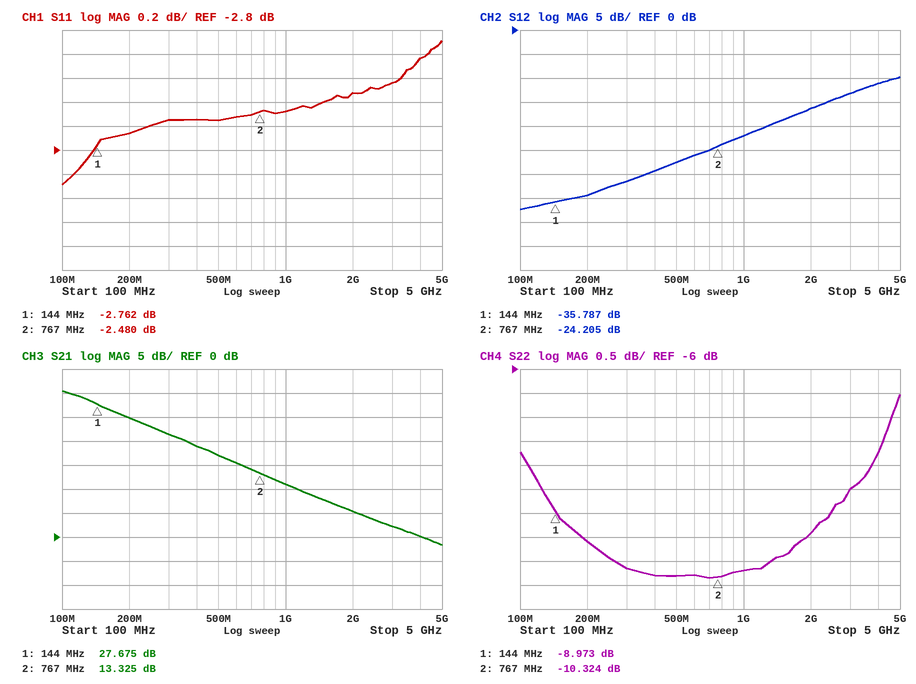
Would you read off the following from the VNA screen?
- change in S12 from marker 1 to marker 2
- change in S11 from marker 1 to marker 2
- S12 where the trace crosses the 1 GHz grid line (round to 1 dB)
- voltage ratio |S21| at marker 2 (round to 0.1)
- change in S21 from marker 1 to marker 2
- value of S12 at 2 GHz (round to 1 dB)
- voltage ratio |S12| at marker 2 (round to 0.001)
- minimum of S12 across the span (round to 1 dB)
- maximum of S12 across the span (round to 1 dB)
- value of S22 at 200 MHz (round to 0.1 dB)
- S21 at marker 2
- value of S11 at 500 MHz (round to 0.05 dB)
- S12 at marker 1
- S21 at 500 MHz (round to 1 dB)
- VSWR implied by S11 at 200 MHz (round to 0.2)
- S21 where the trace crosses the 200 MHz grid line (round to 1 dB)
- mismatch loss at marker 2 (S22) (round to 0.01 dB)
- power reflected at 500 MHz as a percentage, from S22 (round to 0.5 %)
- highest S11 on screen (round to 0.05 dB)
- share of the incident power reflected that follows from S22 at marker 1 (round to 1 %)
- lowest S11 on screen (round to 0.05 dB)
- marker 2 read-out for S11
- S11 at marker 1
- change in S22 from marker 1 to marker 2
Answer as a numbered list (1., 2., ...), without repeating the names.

1. 11.582 dB
2. 0.282 dB
3. -22 dB
4. 4.6
5. -14.350 dB
6. -16 dB
7. 0.062
8. -37 dB
9. -10 dB
10. -9.6 dB
11. 13.325 dB
12. -2.55 dB
13. -35.787 dB
14. 17 dB
15. 6.6
16. 25 dB
17. 0.42 dB
18. 9.5 %
19. -1.90 dB
20. 13 %
21. -3.10 dB
22. -2.480 dB
23. -2.762 dB
24. -1.351 dB
